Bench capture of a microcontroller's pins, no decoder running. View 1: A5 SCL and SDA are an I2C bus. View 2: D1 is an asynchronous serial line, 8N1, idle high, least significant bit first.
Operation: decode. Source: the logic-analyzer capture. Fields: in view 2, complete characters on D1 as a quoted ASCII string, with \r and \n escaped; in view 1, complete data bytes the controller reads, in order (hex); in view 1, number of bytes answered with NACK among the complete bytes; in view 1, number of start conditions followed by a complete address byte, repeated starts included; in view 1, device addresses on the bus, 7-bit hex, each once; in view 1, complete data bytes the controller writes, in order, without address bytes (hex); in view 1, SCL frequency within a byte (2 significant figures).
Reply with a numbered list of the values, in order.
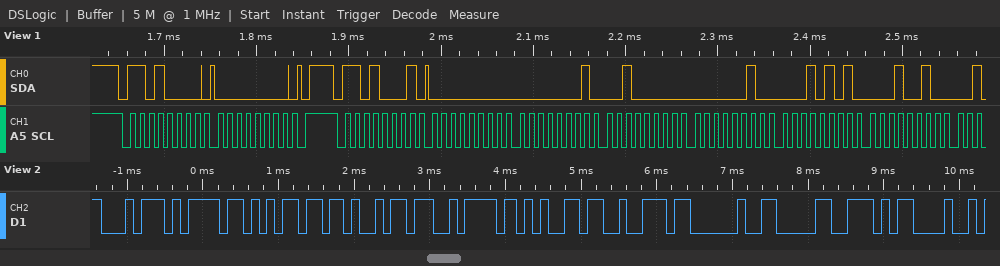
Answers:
1. "tomizer 0\r"
2. 00 01 20 02 15 12
3. 0
4. 2
5. 0x68
6. 00
7. 100 kHz
